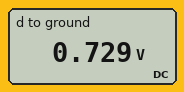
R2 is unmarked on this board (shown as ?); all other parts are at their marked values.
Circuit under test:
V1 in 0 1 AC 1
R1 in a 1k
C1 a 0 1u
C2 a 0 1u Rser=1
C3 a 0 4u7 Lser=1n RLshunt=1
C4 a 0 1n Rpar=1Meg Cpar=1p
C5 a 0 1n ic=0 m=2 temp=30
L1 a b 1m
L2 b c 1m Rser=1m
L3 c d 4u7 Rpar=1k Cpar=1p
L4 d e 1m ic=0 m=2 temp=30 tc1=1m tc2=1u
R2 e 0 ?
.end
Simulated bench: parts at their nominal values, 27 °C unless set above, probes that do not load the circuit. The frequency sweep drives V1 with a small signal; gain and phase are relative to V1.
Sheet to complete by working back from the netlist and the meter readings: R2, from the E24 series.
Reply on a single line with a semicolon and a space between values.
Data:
2.7 kΩ
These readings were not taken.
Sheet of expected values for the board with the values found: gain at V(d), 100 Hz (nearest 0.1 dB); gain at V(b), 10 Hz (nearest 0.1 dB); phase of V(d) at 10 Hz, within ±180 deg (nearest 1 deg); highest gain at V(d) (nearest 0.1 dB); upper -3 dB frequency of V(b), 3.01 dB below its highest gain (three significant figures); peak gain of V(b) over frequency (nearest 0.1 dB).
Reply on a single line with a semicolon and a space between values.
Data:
-12.9 dB; -3.1 dB; -17 deg; -2.7 dB; 32.6 Hz; -2.7 dB
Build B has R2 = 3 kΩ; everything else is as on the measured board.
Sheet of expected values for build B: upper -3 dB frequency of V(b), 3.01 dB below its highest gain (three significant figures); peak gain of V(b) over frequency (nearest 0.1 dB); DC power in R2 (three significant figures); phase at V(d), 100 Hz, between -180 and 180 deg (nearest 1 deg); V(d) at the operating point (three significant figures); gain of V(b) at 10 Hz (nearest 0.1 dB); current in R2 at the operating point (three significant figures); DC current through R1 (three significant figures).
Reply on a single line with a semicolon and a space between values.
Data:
31.7 Hz; -2.5 dB; 187 µW; -72 deg; 749 mV; -2.9 dB; 250 µA; 251 µA
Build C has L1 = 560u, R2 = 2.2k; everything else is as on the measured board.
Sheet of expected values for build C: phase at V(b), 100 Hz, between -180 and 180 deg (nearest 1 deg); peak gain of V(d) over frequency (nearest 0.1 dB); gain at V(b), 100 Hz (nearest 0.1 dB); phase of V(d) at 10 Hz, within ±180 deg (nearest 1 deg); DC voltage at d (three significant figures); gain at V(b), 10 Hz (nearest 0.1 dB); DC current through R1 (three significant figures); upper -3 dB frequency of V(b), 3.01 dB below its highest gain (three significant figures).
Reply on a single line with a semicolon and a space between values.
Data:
-71 deg; -3.3 dB; -13.0 dB; -16 deg; 687 mV; -3.6 dB; 313 µA; 34.6 Hz
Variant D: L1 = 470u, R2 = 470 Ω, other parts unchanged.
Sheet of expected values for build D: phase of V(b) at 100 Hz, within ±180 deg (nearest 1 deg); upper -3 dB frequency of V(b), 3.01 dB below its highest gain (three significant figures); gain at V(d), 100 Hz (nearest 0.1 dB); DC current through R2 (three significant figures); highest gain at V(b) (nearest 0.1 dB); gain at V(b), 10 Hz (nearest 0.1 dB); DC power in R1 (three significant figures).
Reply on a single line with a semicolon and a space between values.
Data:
-53 deg; 74.4 Hz; -14.4 dB; 680 µA; -9.9 dB; -10.0 dB; 463 µW
